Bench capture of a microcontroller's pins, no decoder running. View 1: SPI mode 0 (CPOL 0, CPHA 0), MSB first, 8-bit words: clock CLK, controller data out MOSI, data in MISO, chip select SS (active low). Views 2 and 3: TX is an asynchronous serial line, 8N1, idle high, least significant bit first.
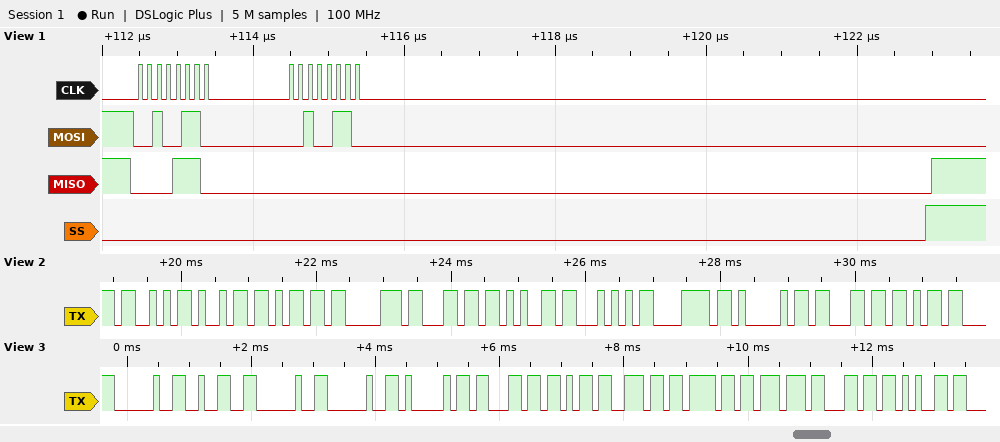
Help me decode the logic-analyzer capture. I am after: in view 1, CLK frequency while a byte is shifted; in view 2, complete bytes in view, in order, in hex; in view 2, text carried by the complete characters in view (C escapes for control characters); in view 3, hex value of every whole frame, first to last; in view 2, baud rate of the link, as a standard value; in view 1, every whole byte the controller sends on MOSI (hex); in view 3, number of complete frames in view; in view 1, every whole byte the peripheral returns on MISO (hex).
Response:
8 MHz
0x53 0x69 0x6D 0x70 0x6C 0x65 0x54 0x78 0x41 0x63 0x6B
"SimpleTxAck"
20 32 20 20 41 63 6B 6E 6F 77 6C 65
9600 baud
0x26 0x26
12
0x0E 0x00
